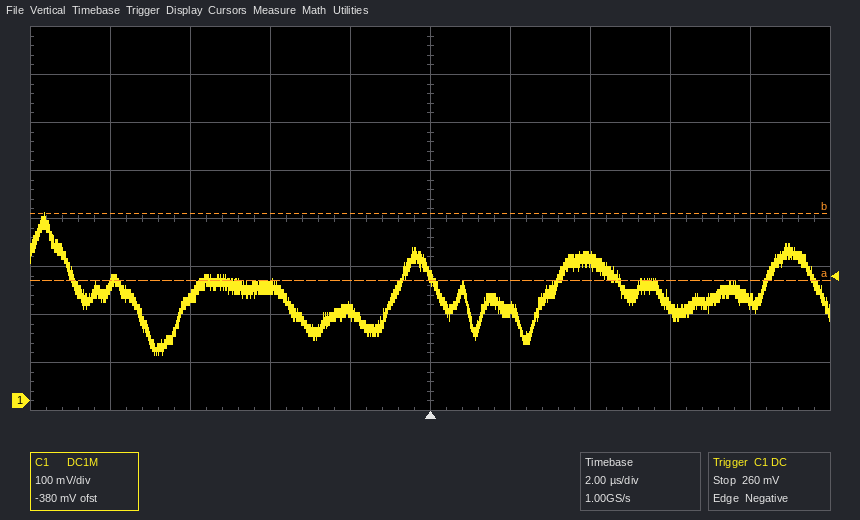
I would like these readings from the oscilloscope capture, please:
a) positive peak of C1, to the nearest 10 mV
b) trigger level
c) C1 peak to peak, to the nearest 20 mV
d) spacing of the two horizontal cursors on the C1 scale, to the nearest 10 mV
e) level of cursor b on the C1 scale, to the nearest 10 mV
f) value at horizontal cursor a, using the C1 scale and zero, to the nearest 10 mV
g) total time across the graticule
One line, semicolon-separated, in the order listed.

390 mV; 260 mV; 300 mV; 140 mV; 390 mV; 250 mV; 20 µs
